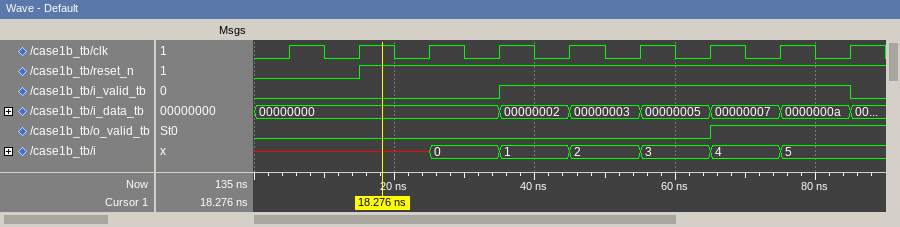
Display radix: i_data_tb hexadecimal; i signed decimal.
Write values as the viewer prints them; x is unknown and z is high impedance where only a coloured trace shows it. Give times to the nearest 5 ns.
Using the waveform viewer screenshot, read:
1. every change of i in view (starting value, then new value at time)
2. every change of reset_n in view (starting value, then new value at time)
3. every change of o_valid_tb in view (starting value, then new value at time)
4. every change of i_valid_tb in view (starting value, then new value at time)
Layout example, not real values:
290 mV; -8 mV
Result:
x, 0 at 25 ns, 1 at 35 ns, 2 at 45 ns, 3 at 55 ns, 4 at 65 ns, 5 at 75 ns; 0, 1 at 15 ns; 0, 1 at 65 ns; 0, 1 at 35 ns, 0 at 85 ns
